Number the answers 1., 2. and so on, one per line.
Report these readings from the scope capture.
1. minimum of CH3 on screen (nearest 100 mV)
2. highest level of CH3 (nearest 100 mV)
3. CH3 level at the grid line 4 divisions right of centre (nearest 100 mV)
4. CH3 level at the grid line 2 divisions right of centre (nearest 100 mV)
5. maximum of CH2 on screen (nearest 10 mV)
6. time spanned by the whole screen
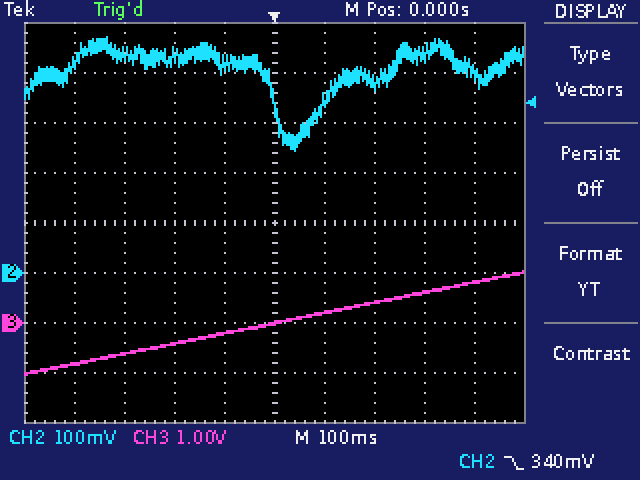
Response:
1. -1.0 V
2. 1.0 V
3. 800 mV
4. 400 mV
5. 470 mV
6. 1 s
